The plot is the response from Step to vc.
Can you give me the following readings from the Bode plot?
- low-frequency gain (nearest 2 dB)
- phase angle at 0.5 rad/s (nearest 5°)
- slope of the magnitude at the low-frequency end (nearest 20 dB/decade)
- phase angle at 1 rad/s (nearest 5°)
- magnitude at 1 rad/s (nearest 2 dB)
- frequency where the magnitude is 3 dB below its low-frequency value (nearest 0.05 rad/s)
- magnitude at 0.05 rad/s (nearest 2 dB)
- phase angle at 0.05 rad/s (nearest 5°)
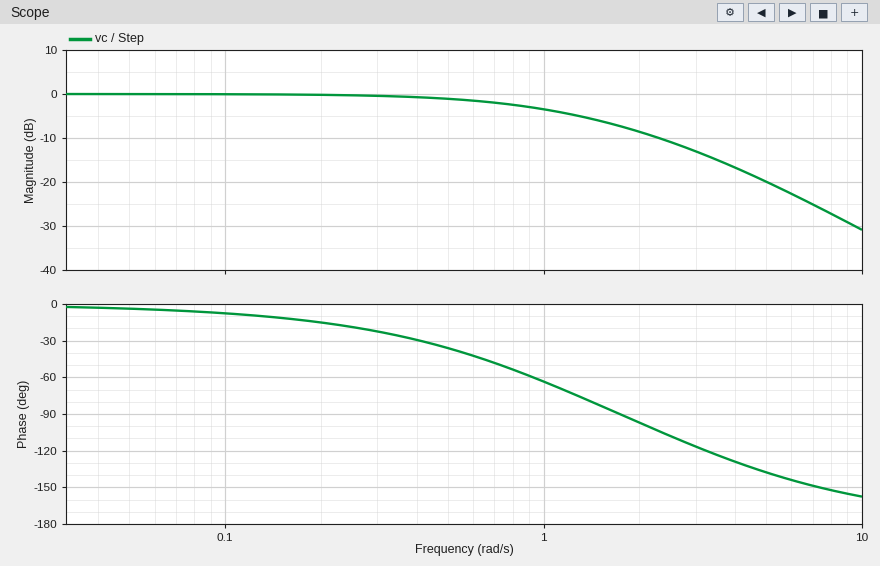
0 dB
-35°
0 dB/decade
-65°
-4 dB
0.90 rad/s
0 dB
-5°
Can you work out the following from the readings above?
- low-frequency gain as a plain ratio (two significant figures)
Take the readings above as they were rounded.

1.0
